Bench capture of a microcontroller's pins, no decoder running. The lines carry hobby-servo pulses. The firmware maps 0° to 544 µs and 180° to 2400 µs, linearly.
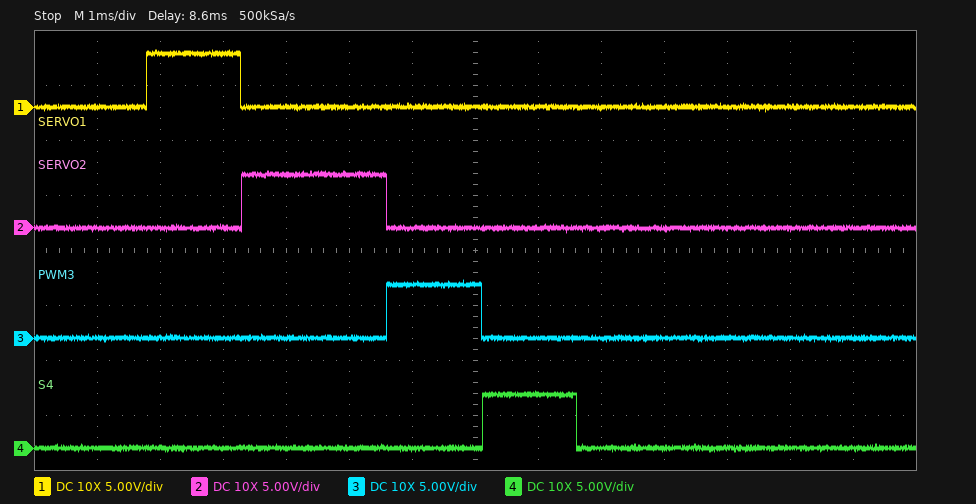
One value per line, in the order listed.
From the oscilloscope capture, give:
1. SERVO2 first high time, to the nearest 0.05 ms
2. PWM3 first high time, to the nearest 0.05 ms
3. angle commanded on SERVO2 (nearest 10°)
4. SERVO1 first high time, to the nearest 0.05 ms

2.30 ms
1.50 ms
170°
1.50 ms
